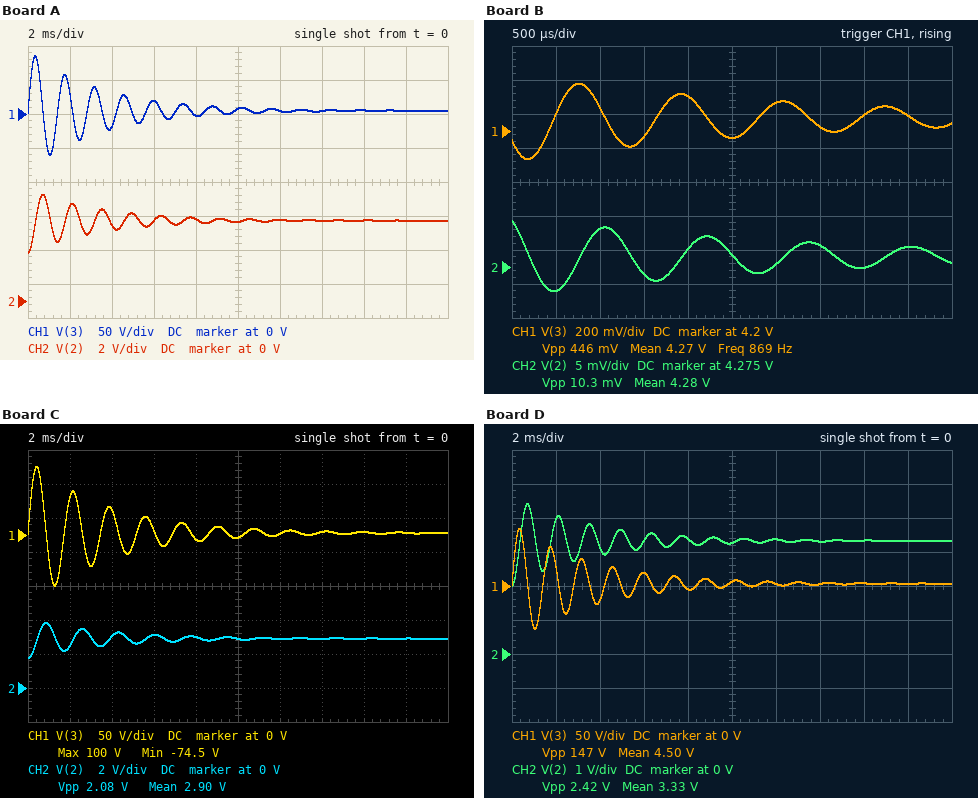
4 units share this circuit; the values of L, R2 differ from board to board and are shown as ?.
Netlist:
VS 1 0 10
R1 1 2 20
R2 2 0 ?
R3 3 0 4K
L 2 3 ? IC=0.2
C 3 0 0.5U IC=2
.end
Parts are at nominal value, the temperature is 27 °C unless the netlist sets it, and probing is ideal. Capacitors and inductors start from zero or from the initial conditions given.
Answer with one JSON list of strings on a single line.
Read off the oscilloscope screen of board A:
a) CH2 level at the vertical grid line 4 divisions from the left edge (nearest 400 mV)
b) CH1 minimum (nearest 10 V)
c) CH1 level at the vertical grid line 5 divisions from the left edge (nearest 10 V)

["4.8 V", "-60 V", "10 V"]
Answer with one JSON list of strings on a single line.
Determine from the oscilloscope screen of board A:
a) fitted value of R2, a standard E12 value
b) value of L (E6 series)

["18 Ω", "100 mH"]
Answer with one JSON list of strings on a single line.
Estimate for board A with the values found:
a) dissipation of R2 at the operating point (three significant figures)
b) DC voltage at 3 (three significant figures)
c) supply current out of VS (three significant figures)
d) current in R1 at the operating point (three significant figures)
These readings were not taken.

["1.24 W", "4.73 V", "264 mA", "264 mA"]
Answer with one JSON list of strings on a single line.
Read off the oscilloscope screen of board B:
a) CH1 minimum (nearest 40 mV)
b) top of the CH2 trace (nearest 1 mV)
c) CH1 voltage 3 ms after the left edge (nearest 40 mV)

["4.04 V", "4.282 V", "4.36 V"]
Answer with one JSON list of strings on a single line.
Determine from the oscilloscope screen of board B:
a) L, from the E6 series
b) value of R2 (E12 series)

["68 mH", "15 Ω"]
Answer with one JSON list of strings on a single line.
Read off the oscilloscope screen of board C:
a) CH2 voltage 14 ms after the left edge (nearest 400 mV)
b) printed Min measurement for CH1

["2.8 V", "-74.5 V"]
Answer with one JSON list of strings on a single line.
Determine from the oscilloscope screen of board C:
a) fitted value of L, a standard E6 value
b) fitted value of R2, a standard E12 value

["150 mH", "8.2 Ω"]
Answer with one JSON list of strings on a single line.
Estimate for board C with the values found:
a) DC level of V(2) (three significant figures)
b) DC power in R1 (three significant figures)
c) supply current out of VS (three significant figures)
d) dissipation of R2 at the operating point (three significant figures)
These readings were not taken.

["2.90 V", "2.52 W", "355 mA", "1.03 W"]
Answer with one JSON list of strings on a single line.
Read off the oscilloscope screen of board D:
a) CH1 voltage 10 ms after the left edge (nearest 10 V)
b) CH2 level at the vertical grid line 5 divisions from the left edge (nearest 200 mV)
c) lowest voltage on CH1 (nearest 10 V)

["10 V", "3.2 V", "-60 V"]
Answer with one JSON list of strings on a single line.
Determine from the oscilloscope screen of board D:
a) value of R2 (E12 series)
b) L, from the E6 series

["10 Ω", "100 mH"]
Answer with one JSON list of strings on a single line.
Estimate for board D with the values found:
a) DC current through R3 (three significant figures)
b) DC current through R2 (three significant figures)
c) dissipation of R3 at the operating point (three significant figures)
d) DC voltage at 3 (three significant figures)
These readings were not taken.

["832 µA", "333 mA", "2.77 mW", "3.33 V"]
